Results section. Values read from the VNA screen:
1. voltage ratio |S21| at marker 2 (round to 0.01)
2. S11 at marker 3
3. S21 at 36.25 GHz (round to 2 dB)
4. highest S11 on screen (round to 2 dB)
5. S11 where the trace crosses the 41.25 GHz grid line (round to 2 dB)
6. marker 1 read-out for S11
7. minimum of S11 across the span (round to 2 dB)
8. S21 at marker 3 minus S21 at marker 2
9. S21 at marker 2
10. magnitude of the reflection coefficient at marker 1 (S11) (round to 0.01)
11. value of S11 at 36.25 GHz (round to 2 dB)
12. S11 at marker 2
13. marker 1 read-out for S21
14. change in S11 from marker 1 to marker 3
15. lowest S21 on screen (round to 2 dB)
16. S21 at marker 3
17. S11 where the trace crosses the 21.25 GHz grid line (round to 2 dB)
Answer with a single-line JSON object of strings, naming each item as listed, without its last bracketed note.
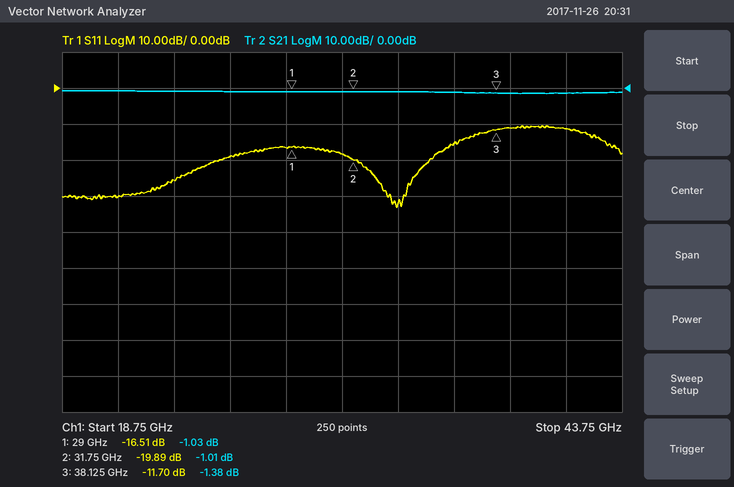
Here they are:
{"voltage ratio |S21| at marker 2": "0.89", "S11 at marker 3": "-11.70 dB", "S21 at 36.25 GHz": "-2 dB", "highest S11 on screen": "-10 dB", "S11 where the trace crosses the 41.25 GHz grid line": "-12 dB", "marker 1 read-out for S11": "-16.51 dB", "minimum of S11 across the span": "-34 dB", "S21 at marker 3 minus S21 at marker 2": "-0.37 dB", "S21 at marker 2": "-1.01 dB", "magnitude of the reflection coefficient at marker 1 (S11)": "0.15", "value of S11 at 36.25 GHz": "-16 dB", "S11 at marker 2": "-19.89 dB", "marker 1 read-out for S21": "-1.03 dB", "change in S11 from marker 1 to marker 3": "4.81 dB", "lowest S21 on screen": "-2 dB", "S21 at marker 3": "-1.38 dB", "S11 where the trace crosses the 21.25 GHz grid line": "-30 dB"}
